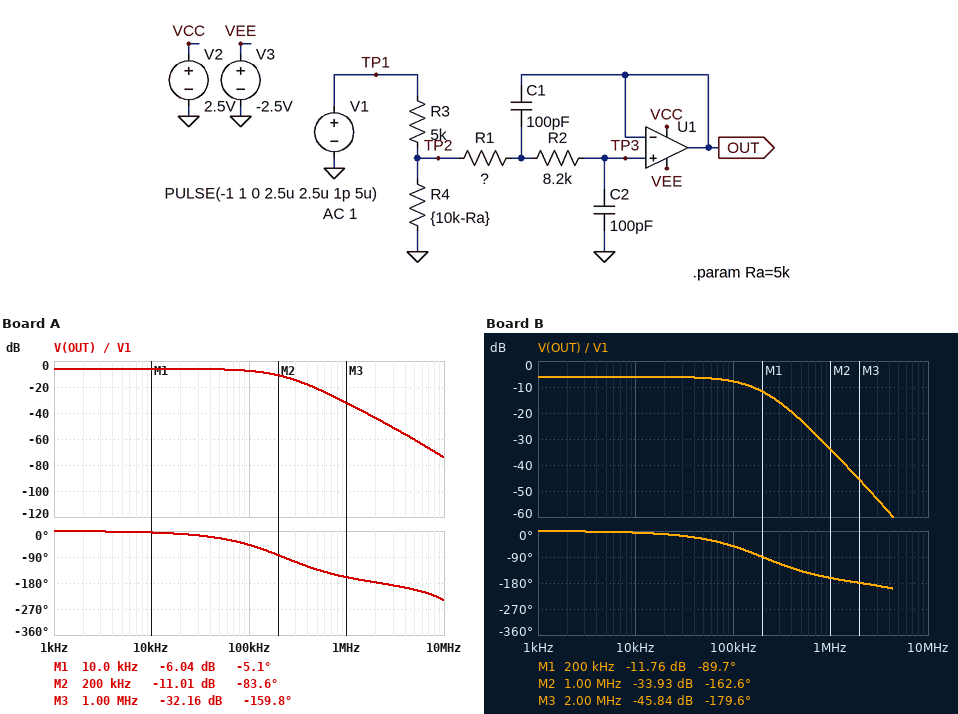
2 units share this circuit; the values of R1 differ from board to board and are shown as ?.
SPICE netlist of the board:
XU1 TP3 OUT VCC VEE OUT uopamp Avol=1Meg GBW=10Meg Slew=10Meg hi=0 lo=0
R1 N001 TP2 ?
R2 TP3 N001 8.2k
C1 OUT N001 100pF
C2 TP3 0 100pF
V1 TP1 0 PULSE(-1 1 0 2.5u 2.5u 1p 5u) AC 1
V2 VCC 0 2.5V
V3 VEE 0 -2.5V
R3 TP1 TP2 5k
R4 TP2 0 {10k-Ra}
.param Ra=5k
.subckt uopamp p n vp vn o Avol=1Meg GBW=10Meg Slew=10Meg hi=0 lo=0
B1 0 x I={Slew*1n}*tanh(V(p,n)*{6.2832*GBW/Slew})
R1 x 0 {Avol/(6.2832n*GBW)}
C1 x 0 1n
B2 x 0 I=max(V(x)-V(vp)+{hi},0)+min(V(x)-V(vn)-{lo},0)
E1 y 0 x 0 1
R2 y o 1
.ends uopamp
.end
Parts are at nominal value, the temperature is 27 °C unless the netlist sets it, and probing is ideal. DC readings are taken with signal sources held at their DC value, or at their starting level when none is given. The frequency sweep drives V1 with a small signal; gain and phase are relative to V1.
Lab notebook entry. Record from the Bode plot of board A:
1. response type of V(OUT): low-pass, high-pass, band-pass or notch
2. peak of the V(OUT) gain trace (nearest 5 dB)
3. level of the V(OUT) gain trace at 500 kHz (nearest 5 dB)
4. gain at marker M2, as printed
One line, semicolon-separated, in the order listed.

low-pass; -5 dB; -20 dB; -11.01 dB
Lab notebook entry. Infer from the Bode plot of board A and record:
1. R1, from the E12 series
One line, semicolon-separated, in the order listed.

3.3 kΩ
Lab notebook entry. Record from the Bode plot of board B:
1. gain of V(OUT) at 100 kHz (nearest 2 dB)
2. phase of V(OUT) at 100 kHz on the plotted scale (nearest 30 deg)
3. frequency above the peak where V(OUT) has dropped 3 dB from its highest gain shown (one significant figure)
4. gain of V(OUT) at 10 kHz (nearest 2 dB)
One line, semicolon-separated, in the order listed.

-8 dB; -60 deg; 100 kHz; -6 dB
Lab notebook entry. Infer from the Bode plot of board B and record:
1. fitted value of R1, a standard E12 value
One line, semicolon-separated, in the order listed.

4.7 kΩ
